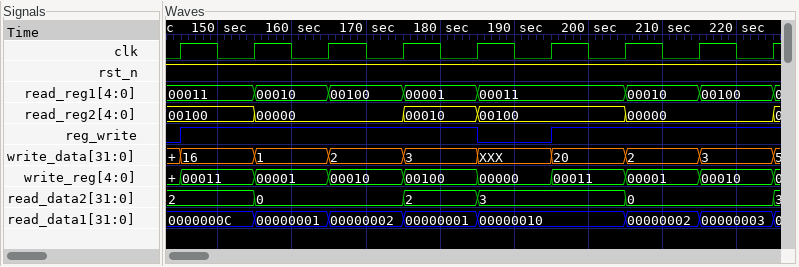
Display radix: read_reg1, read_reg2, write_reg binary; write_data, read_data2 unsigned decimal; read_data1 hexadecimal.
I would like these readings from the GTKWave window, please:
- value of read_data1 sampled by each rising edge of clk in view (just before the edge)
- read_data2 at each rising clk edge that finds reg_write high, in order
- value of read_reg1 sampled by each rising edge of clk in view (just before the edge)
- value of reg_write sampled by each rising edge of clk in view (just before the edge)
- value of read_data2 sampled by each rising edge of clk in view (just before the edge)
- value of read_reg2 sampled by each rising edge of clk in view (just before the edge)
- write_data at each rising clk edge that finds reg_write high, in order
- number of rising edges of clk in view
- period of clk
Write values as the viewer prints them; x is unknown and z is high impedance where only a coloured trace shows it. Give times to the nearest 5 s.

0000000C, 0000000C, 00000001, 00000002, 00000001, 00000010, 00000010, 00000002, 00000003
2, 0, 0, 2, 3, 0, 0
00011, 00011, 00010, 00100, 00001, 00011, 00011, 00010, 00100
0 1 1 1 1 0 1 1 1
2, 2, 0, 0, 2, 3, 3, 0, 0
00100, 00100, 00000, 00000, 00010, 00100, 00100, 00000, 00000
16, 1, 2, 3, 20, 2, 3
9
10 s
